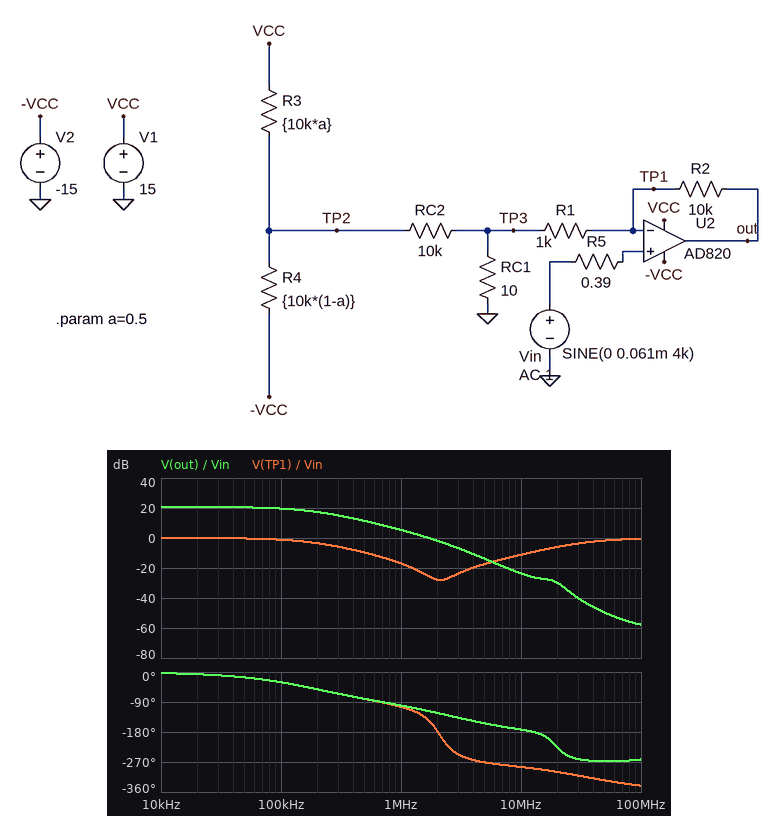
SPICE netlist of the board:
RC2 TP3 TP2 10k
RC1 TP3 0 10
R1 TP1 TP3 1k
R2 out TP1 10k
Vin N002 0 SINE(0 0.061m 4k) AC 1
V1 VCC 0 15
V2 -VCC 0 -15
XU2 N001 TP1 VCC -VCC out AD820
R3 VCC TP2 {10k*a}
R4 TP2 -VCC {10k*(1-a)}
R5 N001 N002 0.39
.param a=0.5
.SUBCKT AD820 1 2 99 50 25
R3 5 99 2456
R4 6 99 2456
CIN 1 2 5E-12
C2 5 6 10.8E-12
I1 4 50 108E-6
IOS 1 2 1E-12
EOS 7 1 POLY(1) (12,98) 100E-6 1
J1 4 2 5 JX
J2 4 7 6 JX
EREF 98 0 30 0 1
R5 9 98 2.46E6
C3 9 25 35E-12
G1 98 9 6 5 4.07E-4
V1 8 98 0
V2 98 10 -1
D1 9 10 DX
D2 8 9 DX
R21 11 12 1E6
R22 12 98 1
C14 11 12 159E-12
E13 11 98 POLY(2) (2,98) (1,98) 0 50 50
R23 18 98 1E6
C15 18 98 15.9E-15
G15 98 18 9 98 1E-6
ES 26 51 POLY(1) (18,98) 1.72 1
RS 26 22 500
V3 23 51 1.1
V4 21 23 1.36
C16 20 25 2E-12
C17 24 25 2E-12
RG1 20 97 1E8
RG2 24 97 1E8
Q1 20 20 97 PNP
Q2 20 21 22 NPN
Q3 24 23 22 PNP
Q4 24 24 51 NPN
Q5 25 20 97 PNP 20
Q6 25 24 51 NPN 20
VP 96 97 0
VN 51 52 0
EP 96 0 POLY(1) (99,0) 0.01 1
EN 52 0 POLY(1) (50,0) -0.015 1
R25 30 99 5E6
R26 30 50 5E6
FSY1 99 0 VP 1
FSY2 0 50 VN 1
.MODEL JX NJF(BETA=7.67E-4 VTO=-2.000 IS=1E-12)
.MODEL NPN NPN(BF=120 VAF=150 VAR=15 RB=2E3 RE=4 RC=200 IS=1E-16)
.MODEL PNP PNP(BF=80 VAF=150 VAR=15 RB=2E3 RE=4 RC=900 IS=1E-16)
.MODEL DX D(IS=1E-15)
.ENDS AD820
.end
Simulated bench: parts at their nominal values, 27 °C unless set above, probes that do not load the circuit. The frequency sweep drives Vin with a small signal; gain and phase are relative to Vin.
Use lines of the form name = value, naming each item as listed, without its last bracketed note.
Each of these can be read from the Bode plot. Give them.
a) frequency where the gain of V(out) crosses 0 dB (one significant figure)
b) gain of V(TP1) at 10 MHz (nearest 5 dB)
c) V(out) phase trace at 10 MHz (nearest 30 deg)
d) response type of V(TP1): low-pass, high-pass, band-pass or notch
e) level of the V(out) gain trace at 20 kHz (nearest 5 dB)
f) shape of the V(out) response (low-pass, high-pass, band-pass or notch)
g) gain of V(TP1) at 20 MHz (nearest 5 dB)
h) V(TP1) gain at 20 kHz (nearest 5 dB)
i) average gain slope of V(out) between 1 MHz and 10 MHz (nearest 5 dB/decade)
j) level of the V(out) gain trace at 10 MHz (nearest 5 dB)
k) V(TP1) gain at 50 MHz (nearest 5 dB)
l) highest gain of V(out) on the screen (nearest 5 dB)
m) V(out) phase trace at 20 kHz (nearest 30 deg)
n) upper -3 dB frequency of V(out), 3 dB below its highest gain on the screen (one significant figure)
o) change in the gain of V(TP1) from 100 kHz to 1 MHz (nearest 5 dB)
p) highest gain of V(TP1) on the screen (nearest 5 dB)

frequency where the gain of V(out) crosses 0 dB = 2 MHz
gain of V(TP1) at 10 MHz = -10 dB
V(out) phase trace at 10 MHz = -180 deg
response type of V(TP1): low-pass, high-pass, band-pass or notch = notch
level of the V(out) gain trace at 20 kHz = 20 dB
shape of the V(out) response = low-pass
gain of V(TP1) at 20 MHz = -5 dB
V(TP1) gain at 20 kHz = 0 dB
average gain slope of V(out) between 1 MHz and 10 MHz = -30 dB/decade
level of the V(out) gain trace at 10 MHz = -25 dB
V(TP1) gain at 50 MHz = 0 dB
highest gain of V(out) on the screen = 20 dB
V(out) phase trace at 20 kHz = 0 deg
upper -3 dB frequency of V(out), 3 dB below its highest gain on the screen = 200 kHz
change in the gain of V(TP1) from 100 kHz to 1 MHz = -15 dB
highest gain of V(TP1) on the screen = 0 dB
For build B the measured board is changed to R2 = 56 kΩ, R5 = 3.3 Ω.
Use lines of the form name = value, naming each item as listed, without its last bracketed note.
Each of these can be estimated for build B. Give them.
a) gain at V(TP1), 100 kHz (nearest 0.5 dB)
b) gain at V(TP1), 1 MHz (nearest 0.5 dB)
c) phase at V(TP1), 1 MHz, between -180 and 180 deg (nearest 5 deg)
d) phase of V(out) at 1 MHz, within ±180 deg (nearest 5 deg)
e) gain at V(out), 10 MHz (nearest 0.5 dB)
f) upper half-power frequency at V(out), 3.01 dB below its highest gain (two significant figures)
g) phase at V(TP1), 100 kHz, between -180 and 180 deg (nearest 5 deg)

gain at V(TP1), 100 kHz = -10.0 dB
gain at V(TP1), 1 MHz = -40.0 dB
phase at V(TP1), 1 MHz, between -180 and 180 deg = 170 deg
phase of V(out) at 1 MHz, within ±180 deg = -110 deg
gain at V(out), 10 MHz = -24.0 dB
upper half-power frequency at V(out), 3.01 dB below its highest gain = 33 kHz
phase at V(TP1), 100 kHz, between -180 and 180 deg = -75 deg
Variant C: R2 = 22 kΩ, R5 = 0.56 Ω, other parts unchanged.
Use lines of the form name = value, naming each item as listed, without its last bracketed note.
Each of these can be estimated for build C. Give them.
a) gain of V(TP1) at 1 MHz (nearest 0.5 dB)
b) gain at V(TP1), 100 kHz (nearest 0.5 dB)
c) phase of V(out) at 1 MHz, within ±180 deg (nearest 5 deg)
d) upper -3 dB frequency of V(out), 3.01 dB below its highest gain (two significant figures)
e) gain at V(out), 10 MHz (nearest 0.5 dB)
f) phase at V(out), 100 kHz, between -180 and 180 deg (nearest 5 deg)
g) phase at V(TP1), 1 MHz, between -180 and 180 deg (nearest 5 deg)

gain of V(TP1) at 1 MHz = -26.0 dB
gain at V(TP1), 100 kHz = -4.0 dB
phase of V(out) at 1 MHz, within ±180 deg = -105 deg
upper -3 dB frequency of V(out), 3.01 dB below its highest gain = 84 kHz
gain at V(out), 10 MHz = -24.0 dB
phase at V(out), 100 kHz, between -180 and 180 deg = -50 deg
phase at V(TP1), 1 MHz, between -180 and 180 deg = -115 deg
